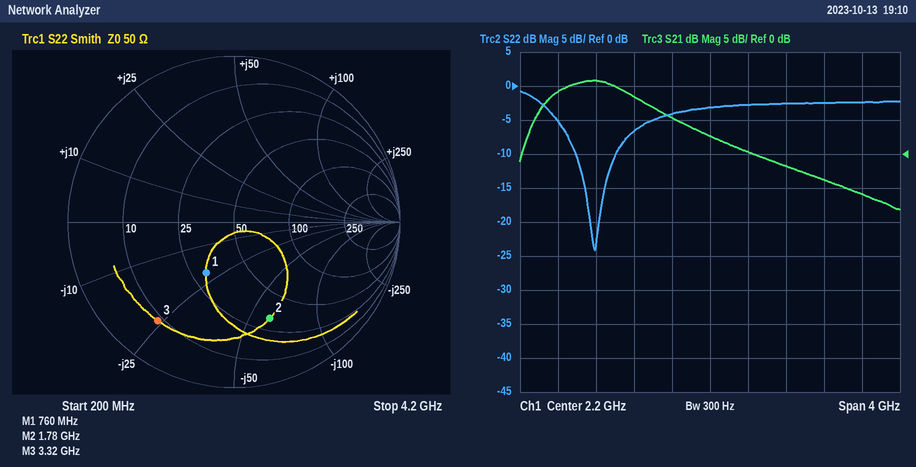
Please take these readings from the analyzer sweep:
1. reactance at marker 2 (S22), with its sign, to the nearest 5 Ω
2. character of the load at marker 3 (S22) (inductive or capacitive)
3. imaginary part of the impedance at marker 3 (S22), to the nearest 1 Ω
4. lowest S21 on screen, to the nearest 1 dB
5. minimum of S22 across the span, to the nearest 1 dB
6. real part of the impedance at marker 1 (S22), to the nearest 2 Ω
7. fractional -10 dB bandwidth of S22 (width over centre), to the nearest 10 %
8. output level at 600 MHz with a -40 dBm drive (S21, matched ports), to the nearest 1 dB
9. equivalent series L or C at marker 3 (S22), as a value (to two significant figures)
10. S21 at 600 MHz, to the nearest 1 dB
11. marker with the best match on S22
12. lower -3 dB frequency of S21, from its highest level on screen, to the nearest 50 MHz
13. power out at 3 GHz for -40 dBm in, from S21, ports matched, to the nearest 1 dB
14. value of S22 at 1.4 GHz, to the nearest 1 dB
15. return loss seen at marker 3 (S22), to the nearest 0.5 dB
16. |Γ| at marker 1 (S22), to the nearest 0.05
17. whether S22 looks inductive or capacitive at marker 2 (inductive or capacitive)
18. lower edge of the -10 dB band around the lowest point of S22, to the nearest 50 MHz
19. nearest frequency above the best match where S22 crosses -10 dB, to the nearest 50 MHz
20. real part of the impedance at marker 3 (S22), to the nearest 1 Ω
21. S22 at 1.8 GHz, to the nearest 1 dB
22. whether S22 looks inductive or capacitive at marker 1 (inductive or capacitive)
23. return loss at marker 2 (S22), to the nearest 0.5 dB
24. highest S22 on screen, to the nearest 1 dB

-60 Ω
capacitive
-24 Ω
-8 dB
-24 dB
30 Ω
40 %
-31 dBm
2.0 pF
9 dB
marker 1
500 MHz
-42 dBm
-7 dB
2.5 dB
0.35
capacitive
800 MHz
1.20 GHz
9 Ω
-4 dB
capacitive
4.0 dB
-1 dB
